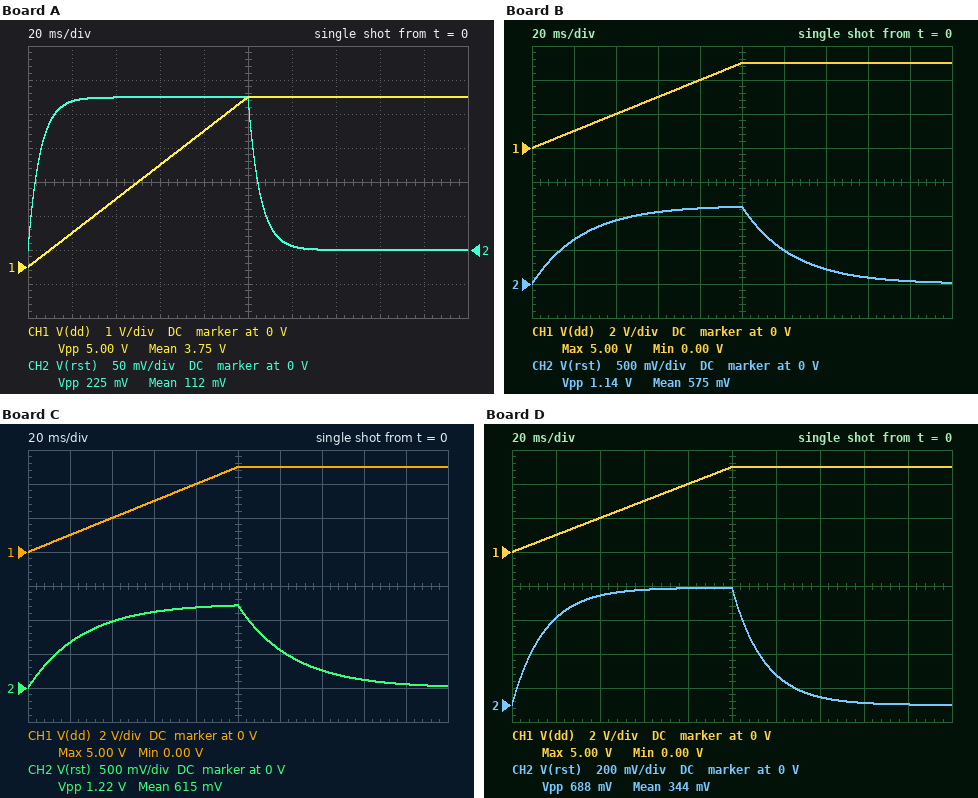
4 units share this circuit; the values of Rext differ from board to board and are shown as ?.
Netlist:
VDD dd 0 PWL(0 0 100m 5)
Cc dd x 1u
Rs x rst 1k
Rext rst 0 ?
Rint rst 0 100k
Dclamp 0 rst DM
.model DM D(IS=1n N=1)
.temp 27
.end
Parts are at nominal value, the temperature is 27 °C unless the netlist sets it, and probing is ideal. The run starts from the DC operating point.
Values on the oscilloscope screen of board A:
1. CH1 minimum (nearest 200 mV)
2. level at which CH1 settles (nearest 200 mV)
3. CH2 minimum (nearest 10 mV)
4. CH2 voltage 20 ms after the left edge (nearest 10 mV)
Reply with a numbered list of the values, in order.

1. 0 V
2. 5.0 V
3. 0 V
4. 220 mV
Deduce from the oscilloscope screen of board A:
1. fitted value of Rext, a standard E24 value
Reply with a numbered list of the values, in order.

1. 4.7 kΩ
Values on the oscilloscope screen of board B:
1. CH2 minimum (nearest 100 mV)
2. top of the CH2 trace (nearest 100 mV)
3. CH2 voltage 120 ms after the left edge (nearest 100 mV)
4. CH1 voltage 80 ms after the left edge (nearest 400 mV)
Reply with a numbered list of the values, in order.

1. 0 V
2. 1.1 V
3. 500 mV
4. 4.0 V
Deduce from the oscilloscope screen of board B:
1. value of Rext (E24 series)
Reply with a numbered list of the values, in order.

1. 30 kΩ
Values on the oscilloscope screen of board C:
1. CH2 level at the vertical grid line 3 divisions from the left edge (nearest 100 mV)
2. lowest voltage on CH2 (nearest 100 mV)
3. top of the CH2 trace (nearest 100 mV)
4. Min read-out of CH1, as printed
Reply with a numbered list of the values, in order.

1. 1.1 V
2. 0 V
3. 1.2 V
4. 0.00 V
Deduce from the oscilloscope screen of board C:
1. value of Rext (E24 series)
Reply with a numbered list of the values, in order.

1. 33 kΩ
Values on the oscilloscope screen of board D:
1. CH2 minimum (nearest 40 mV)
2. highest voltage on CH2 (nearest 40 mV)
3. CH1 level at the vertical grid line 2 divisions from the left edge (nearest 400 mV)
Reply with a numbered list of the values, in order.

1. 0 V
2. 680 mV
3. 2.0 V
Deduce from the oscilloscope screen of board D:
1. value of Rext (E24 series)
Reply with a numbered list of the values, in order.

1. 16 kΩ
